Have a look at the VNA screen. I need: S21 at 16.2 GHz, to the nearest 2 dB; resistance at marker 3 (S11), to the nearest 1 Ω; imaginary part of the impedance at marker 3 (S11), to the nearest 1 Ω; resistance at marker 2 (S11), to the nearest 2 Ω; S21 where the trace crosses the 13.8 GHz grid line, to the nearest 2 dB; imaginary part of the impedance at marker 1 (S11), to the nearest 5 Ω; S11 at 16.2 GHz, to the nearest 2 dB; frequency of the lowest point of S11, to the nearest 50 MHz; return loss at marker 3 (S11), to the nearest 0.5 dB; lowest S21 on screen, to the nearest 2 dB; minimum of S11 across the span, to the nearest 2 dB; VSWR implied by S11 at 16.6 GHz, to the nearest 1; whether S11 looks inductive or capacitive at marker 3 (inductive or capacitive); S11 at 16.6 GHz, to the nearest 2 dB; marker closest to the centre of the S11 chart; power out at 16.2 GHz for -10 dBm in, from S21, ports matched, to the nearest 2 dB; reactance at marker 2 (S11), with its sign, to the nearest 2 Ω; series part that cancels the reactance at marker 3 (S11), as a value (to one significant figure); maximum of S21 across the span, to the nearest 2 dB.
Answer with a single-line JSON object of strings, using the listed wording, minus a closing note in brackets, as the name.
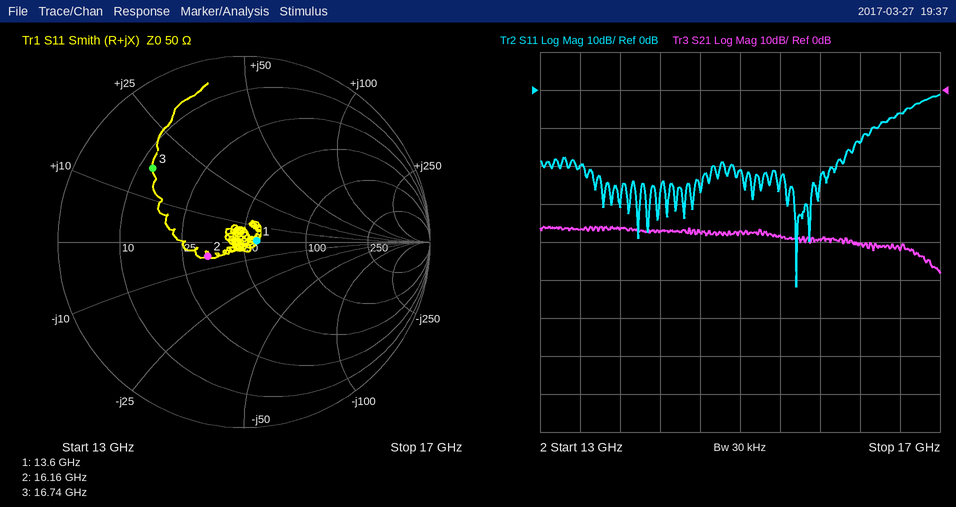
{"S21 at 16.2 GHz, to the nearest 2 dB": "-40 dB", "resistance at marker 3 (S11), to the nearest 1 Ω": "13 Ω", "imaginary part of the impedance at marker 3 (S11), to the nearest 1 Ω": "+17 Ω", "resistance at marker 2 (S11), to the nearest 2 Ω": "34 Ω", "S21 where the trace crosses the 13.8 GHz grid line, to the nearest 2 dB": "-36 dB", "imaginary part of the impedance at marker 1 (S11), to the nearest 5 Ω": "0 Ω", "S11 at 16.2 GHz, to the nearest 2 dB": "-14 dB", "frequency of the lowest point of S11, to the nearest 50 MHz": "15.55 GHz", "return loss at marker 3 (S11), to the nearest 0.5 dB": "4.0 dB", "lowest S21 on screen, to the nearest 2 dB": "-48 dB", "minimum of S11 across the span, to the nearest 2 dB": "-52 dB", "VSWR implied by S11 at 16.6 GHz, to the nearest 1": "3", "whether S11 looks inductive or capacitive at marker 3": "inductive", "S11 at 16.6 GHz, to the nearest 2 dB": "-6 dB", "marker closest to the centre of the S11 chart": "marker 1", "power out at 16.2 GHz for -10 dBm in, from S21, ports matched, to the nearest 2 dB": "-50 dBm", "reactance at marker 2 (S11), with its sign, to the nearest 2 Ω": "-6 Ω", "series part that cancels the reactance at marker 3 (S11), as a value": "600 fF", "maximum of S21 across the span, to the nearest 2 dB": "-36 dB"}
